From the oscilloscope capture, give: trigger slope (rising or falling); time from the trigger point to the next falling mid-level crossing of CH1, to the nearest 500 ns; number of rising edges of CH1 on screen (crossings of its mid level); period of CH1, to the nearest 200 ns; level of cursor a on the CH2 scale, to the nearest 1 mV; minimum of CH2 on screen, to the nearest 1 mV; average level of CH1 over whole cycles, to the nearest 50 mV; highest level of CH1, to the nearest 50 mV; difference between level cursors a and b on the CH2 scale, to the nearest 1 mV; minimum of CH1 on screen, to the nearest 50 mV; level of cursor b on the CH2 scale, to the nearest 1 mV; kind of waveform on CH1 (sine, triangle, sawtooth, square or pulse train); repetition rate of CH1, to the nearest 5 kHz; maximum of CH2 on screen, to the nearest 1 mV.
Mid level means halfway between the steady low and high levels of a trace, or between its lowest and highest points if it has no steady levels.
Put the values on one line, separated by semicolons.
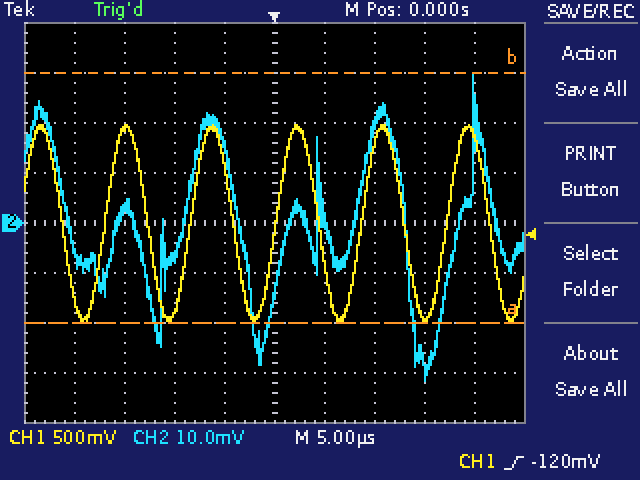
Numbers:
rising; 4.5 µs; 5; 8.6 µs; -20 mV; -32 mV; 0 mV; 1.00 V; 50 mV; -1.00 V; 30 mV; sine; 115 kHz; 30 mV
